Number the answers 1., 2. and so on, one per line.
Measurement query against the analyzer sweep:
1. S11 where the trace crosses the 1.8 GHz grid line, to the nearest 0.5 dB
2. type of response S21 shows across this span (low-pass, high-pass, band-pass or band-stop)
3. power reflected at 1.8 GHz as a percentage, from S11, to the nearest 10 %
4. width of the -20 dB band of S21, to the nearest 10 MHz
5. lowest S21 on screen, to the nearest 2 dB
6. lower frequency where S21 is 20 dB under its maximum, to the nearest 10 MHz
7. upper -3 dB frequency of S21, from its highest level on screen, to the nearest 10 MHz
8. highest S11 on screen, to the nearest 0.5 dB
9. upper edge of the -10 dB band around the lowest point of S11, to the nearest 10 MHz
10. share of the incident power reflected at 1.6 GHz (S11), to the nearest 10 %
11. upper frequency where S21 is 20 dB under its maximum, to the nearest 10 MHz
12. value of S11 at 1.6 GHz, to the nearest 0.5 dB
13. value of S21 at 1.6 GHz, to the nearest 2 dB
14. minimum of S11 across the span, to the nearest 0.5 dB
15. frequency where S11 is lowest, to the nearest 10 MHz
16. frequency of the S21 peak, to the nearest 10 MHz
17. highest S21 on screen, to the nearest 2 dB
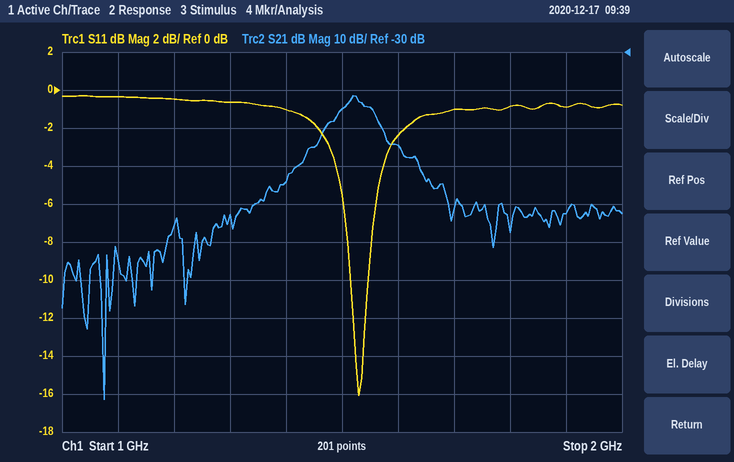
1. -1.0 dB
2. band-pass
3. 80 %
4. 230 MHz
5. -122 dB
6. 1.41 GHz
7. 1.55 GHz
8. -0.5 dB
9. 1.55 GHz
10. 60 %
11. 1.64 GHz
12. -2.5 dB
13. -54 dB
14. -16.0 dB
15. 1.53 GHz
16. 1.52 GHz
17. -42 dB
